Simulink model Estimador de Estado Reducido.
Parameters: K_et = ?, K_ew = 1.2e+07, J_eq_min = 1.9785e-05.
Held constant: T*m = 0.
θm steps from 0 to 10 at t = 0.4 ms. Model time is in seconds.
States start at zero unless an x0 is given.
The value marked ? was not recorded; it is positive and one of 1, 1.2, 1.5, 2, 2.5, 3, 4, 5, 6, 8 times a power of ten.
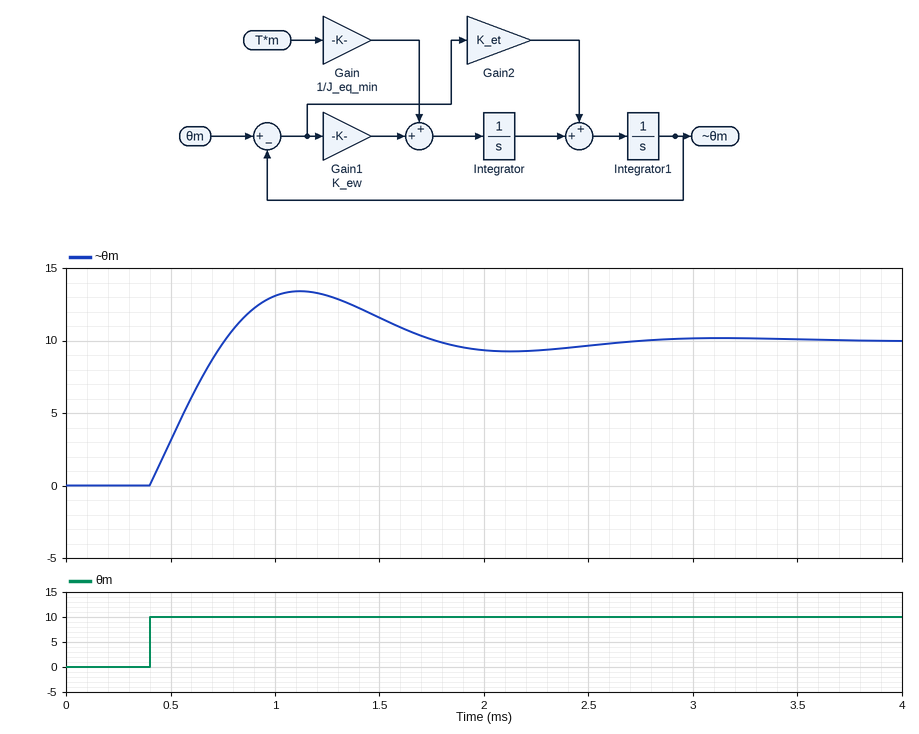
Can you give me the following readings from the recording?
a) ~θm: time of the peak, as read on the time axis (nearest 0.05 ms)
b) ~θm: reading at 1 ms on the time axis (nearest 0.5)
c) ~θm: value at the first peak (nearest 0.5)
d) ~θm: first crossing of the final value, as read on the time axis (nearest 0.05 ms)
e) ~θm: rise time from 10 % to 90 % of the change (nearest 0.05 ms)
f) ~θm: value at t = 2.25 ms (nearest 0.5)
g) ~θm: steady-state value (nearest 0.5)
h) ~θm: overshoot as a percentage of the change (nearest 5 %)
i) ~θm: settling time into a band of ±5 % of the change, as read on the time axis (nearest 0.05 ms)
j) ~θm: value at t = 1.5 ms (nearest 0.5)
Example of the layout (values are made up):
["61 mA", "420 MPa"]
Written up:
["1.10 ms", "13.0", "13.5", "0.75 ms", "0.30 ms", "9.5", "10.0", "35 %", "2.40 ms", "11.5"]
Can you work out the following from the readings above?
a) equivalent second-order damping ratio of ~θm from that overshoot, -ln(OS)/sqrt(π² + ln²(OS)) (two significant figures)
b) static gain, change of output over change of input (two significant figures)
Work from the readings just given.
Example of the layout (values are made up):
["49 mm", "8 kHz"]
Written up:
["0.32", "1.0"]
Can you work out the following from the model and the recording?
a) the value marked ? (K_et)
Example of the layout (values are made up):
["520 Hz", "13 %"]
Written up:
["3000"]
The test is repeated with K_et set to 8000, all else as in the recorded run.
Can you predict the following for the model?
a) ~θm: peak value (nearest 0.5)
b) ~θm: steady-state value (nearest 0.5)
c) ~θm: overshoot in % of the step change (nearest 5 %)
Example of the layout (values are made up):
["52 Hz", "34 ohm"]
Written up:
["11.0", "10.0", "10 %"]
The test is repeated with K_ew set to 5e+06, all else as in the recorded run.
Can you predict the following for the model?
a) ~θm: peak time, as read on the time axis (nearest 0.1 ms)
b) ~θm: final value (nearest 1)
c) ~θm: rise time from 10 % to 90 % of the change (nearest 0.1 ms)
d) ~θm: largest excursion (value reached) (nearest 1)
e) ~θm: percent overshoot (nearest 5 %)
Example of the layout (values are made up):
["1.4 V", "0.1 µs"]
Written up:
["1.4 ms", "10", "0.4 ms", "12", "20 %"]
